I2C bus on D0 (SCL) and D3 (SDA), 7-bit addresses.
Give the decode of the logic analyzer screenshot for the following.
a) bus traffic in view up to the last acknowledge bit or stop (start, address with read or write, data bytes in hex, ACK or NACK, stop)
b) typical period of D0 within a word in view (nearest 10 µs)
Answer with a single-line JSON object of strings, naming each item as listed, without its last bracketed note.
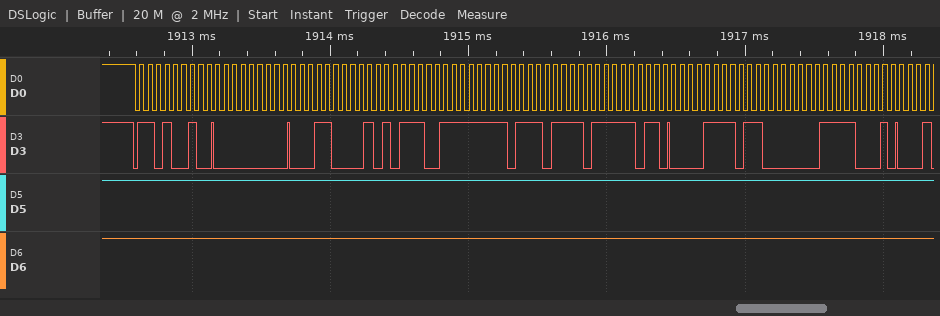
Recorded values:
{"bus traffic in view up to the last acknowledge bit or stop": "start, address 69 write ACK, 00 ACK, 18 ACK, AE ACK, FF ACK, EF ACK, FB ACK, 0F ACK, C0 ACK, F1 ACK", "typical period of D0 within a word in view": "60 µs"}
